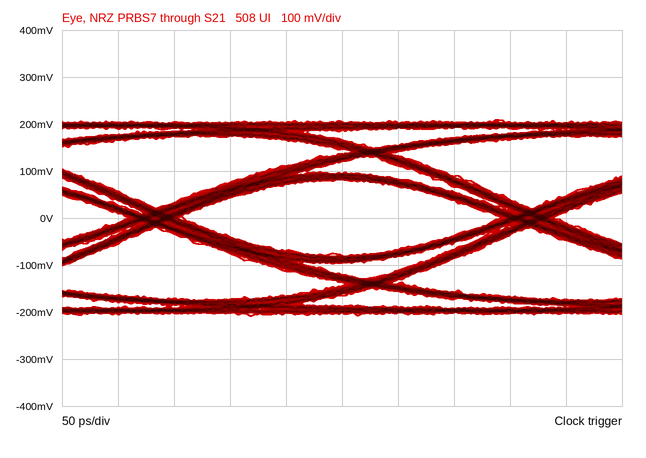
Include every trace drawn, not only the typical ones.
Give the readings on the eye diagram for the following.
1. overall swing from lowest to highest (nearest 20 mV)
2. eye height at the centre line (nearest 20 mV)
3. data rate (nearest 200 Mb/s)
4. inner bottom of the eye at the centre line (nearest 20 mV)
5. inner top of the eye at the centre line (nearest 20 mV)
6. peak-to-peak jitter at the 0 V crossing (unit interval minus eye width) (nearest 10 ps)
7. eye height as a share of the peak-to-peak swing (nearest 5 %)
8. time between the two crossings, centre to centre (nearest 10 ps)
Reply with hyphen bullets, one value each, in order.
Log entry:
- 420 mV
- 160 mV
- 3.0 Gb/s
- -80 mV
- 80 mV
- 50 ps
- 40 %
- 330 ps
